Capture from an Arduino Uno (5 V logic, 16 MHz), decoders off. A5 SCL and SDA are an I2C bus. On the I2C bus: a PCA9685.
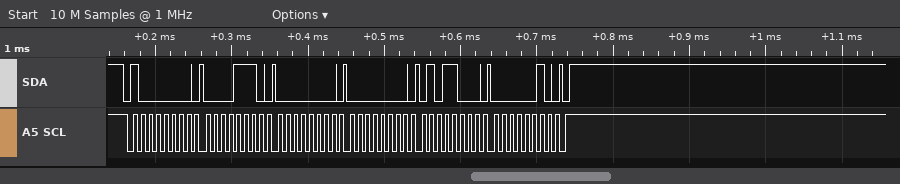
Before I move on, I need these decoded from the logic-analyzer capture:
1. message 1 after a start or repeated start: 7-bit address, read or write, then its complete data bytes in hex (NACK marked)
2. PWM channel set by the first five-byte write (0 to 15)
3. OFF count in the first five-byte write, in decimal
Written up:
0x40 write: 0E 00 00 58 02
2
600
